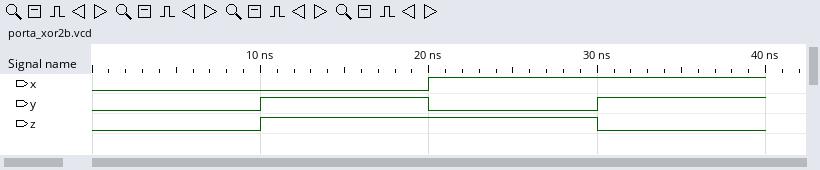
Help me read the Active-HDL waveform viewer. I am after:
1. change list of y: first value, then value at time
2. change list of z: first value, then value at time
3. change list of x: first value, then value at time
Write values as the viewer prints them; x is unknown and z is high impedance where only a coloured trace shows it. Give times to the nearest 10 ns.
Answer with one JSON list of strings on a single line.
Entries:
["0, 1 at 10 ns, 0 at 20 ns, 1 at 30 ns", "0, 1 at 10 ns, 0 at 30 ns", "0, 1 at 20 ns"]
